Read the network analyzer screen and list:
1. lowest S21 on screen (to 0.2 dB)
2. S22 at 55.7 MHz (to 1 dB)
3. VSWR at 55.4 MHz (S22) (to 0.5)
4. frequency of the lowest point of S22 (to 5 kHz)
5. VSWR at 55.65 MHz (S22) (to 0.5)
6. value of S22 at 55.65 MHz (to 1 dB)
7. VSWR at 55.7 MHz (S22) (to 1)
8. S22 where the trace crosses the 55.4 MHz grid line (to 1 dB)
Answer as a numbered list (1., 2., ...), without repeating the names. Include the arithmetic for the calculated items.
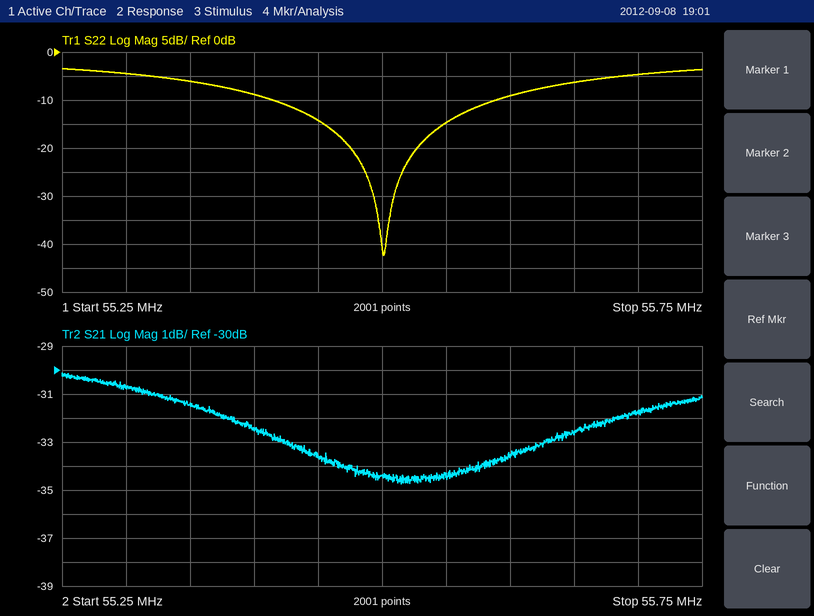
1. -34.8 dB
2. -5 dB
3. |Γ| = 10^(-9/20) = 0.3548; VSWR = (1 + 0.3548)/(1 − 0.3548) ≈ 2.10, so 2.0 to the nearest 0.5
4. 55.500 MHz
5. |Γ| = 10^(-6/20) = 0.5012; VSWR = (1 + 0.5012)/(1 − 0.5012) ≈ 3.0
6. -6 dB
7. |Γ| = 10^(-5/20) = 0.5623; VSWR = (1 + 0.5623)/(1 − 0.5623) ≈ 4
8. -9 dB
